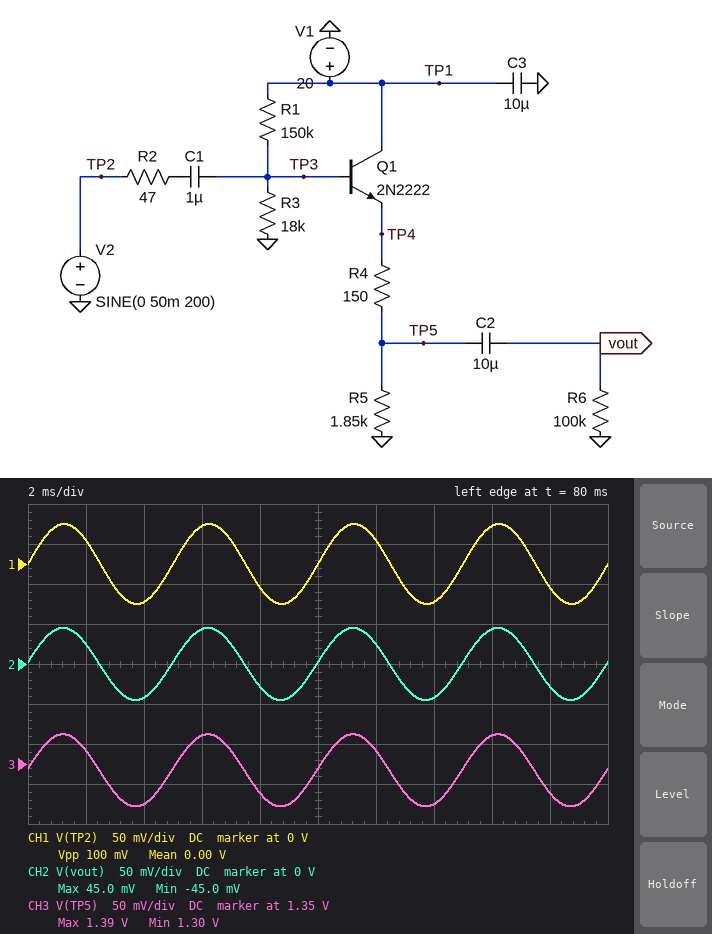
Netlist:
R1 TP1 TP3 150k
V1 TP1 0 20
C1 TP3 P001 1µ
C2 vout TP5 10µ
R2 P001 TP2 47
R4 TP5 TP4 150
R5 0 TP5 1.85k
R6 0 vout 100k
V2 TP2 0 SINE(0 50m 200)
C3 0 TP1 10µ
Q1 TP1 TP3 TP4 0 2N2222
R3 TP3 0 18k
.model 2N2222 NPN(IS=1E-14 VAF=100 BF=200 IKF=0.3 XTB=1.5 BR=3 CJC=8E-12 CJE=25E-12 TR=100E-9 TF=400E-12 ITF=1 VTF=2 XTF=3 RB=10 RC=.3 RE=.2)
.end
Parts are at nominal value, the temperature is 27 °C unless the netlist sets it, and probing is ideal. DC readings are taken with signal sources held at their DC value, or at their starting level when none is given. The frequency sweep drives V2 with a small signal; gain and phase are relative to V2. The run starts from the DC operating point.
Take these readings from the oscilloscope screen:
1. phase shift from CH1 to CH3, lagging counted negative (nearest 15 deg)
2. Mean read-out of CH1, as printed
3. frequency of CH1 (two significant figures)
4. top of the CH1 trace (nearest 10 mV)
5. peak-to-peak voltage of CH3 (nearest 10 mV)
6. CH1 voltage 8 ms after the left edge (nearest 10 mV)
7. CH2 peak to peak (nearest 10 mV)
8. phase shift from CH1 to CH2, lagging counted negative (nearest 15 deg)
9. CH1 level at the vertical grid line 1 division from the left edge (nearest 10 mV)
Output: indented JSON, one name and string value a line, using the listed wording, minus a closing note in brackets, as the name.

{
  "phase shift from CH1 to CH3, lagging counted negative": "0 deg",
  "Mean read-out of CH1, as printed": "0.00 V",
  "frequency of CH1": "200 Hz",
  "top of the CH1 trace": "50 mV",
  "peak-to-peak voltage of CH3": "90 mV",
  "CH1 voltage 8 ms after the left edge": "-30 mV",
  "CH2 peak to peak": "90 mV",
  "phase shift from CH1 to CH2, lagging counted negative": "0 deg",
  "CH1 level at the vertical grid line 1 division from the left edge": "30 mV"
}
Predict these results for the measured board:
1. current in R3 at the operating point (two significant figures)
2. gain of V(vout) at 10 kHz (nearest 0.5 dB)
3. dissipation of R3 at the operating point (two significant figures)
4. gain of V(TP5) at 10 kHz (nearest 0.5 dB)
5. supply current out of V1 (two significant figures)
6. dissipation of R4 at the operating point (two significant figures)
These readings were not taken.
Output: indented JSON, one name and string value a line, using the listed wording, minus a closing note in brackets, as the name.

{
  "current in R3 at the operating point": "120 µA",
  "gain of V(vout) at 10 kHz": "-1.0 dB",
  "dissipation of R3 at the operating point": "240 µW",
  "gain of V(TP5) at 10 kHz": "-1.0 dB",
  "supply current out of V1": "840 µA",
  "dissipation of R4 at the operating point": "79 µW"
}
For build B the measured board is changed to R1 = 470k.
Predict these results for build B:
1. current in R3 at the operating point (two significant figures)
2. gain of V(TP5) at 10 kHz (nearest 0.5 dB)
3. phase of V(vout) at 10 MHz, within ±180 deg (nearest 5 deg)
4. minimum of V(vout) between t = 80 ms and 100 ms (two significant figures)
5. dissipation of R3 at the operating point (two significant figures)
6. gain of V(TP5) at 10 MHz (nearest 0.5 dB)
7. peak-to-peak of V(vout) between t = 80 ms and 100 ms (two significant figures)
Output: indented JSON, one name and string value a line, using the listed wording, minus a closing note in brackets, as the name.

{
  "current in R3 at the operating point": "41 µA",
  "gain of V(TP5) at 10 kHz": "-2.0 dB",
  "phase of V(vout) at 10 MHz, within ±180 deg": "5 deg",
  "minimum of V(vout) between t = 80 ms and 100 ms": "-38 mV",
  "dissipation of R3 at the operating point": "30 µW",
  "gain of V(TP5) at 10 MHz": "-1.5 dB",
  "peak-to-peak of V(vout) between t = 80 ms and 100 ms": "78 mV"
}
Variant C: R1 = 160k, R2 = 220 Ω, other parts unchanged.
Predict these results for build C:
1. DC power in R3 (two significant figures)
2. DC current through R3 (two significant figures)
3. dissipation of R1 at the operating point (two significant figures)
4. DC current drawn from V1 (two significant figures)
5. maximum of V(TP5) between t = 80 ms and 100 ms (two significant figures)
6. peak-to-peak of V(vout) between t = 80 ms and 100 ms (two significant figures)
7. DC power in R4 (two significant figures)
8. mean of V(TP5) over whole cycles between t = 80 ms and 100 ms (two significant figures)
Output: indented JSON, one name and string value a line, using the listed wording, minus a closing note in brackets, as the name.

{
  "DC power in R3": "220 µW",
  "DC current through R3": "110 µA",
  "dissipation of R1 at the operating point": "2.0 mW",
  "DC current drawn from V1": "780 µA",
  "maximum of V(TP5) between t = 80 ms and 100 ms": "1.3 V",
  "peak-to-peak of V(vout) between t = 80 ms and 100 ms": "89 mV",
  "DC power in R4": "67 µW",
  "mean of V(TP5) over whole cycles between t = 80 ms and 100 ms": "1.2 V"
}
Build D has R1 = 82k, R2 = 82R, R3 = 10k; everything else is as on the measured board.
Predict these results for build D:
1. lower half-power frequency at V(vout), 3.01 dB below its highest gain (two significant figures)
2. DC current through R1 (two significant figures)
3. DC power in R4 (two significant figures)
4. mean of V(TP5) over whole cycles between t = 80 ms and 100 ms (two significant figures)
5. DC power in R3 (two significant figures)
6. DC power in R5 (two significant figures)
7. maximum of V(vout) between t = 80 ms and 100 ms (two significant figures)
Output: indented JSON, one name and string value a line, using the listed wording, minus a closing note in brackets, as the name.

{
  "lower half-power frequency at V(vout), 3.01 dB below its highest gain": "18 Hz",
  "DC current through R1": "220 µA",
  "DC power in R4": "85 µW",
  "mean of V(TP5) over whole cycles between t = 80 ms and 100 ms": "1.4 V",
  "DC power in R3": "460 µW",
  "DC power in R5": "1.0 mW",
  "maximum of V(vout) between t = 80 ms and 100 ms": "45 mV"
}
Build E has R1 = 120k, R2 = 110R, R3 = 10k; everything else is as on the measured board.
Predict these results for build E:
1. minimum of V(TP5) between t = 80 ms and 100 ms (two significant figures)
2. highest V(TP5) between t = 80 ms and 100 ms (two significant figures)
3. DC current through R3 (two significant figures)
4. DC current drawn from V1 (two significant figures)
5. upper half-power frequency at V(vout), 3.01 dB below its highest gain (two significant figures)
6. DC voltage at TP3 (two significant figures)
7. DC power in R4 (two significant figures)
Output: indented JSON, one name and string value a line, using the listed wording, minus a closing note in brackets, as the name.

{
  "minimum of V(TP5) between t = 80 ms and 100 ms": "780 mV",
  "highest V(TP5) between t = 80 ms and 100 ms": "870 mV",
  "DC current through R3": "150 µA",
  "DC current drawn from V1": "600 µA",
  "upper half-power frequency at V(vout), 3.01 dB below its highest gain": "480 MHz",
  "DC voltage at TP3": "1.5 V",
  "DC power in R4": "30 µW"
}
